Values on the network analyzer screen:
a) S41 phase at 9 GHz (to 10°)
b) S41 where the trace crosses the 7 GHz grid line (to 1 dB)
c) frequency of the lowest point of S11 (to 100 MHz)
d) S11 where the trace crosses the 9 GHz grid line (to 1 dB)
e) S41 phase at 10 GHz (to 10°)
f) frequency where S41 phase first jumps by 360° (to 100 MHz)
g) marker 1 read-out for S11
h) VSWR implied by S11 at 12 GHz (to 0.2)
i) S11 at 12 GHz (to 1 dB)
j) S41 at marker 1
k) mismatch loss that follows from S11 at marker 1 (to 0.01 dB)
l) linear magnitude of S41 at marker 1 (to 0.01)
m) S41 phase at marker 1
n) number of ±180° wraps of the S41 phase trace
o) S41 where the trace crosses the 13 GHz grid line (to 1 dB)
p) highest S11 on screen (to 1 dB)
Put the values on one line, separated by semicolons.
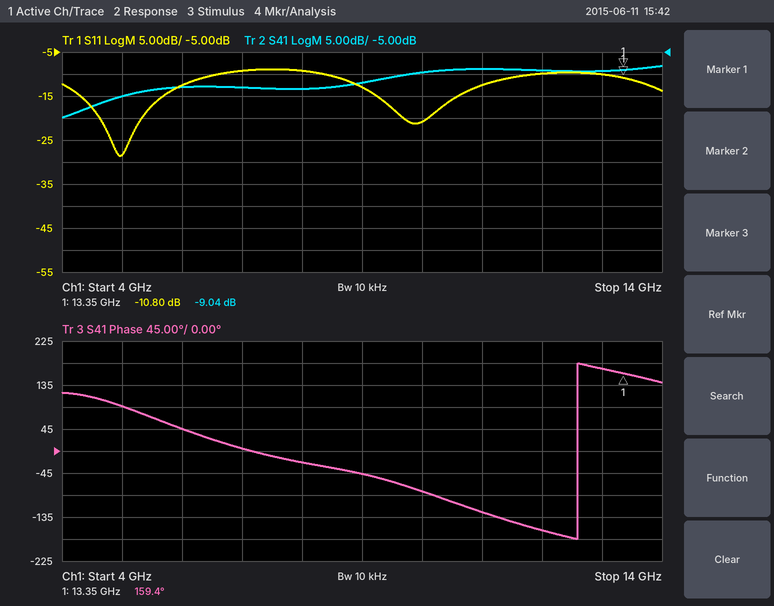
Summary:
-50°; -13 dB; 5.0 GHz; -13 dB; -80°; 12.6 GHz; -10.80 dB; 2.0; -10 dB; -9.04 dB; 0.38 dB; 0.35; 159.4°; 1; -9 dB; -9 dB
